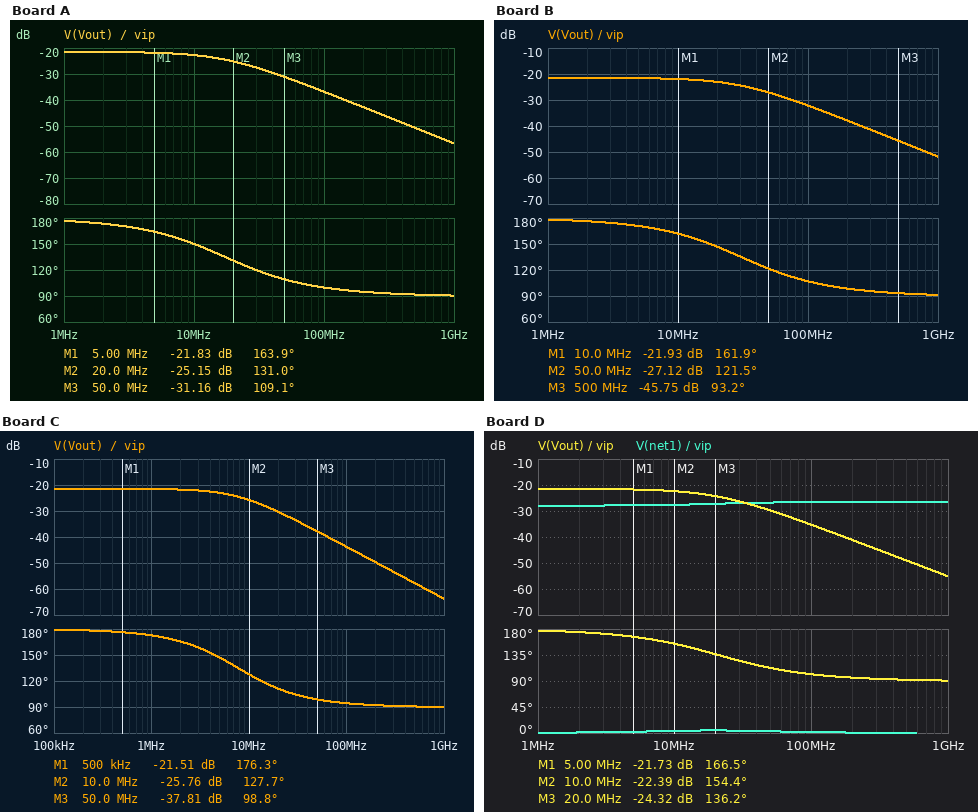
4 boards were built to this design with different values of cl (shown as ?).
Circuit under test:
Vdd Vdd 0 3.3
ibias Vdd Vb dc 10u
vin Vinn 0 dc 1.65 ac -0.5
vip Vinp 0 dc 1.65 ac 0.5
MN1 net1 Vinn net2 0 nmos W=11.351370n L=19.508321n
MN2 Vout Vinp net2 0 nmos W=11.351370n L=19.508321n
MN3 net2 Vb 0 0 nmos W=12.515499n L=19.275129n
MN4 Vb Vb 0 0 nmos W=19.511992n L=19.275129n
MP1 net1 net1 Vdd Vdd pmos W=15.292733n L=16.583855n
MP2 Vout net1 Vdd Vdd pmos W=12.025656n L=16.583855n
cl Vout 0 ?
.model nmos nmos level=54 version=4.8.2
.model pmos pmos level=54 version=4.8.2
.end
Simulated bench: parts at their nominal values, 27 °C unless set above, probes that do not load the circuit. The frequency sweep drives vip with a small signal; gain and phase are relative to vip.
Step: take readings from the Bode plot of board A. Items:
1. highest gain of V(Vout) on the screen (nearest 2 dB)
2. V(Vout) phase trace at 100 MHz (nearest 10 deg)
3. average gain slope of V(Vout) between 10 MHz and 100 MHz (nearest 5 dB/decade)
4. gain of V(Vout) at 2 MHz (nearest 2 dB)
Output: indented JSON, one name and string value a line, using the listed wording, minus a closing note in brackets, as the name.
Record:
{
  "highest gain of V(Vout) on the screen": "-22 dB",
  "V(Vout) phase trace at 100 MHz": "100 deg",
  "average gain slope of V(Vout) between 10 MHz and 100 MHz": "-15 dB/decade",
  "gain of V(Vout) at 2 MHz": "-22 dB"
}
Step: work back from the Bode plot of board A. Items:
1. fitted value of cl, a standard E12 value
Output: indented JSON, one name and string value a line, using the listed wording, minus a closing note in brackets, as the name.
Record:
{
  "fitted value of cl, a standard E12 value": "1.2 pF"
}
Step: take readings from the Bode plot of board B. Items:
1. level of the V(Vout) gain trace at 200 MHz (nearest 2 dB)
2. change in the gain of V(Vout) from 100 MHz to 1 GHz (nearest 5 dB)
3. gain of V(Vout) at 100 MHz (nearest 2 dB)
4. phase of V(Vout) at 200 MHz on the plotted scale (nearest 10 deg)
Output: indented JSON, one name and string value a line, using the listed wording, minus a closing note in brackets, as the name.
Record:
{
  "level of the V(Vout) gain trace at 200 MHz": "-38 dB",
  "change in the gain of V(Vout) from 100 MHz to 1 GHz": "-20 dB",
  "gain of V(Vout) at 100 MHz": "-32 dB",
  "phase of V(Vout) at 200 MHz on the plotted scale": "100 deg"
}
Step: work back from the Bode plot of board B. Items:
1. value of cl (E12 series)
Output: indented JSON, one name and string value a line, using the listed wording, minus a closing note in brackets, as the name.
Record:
{
  "value of cl": "680 fF"
}
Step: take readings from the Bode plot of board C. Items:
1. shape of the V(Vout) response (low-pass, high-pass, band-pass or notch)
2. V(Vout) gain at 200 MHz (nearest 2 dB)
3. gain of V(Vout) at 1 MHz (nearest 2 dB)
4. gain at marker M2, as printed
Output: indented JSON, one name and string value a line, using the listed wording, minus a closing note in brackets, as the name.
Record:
{
  "shape of the V(Vout) response": "low-pass",
  "V(Vout) gain at 200 MHz": "-50 dB",
  "gain of V(Vout) at 1 MHz": "-22 dB",
  "gain at marker M2, as printed": "-25.76 dB"
}
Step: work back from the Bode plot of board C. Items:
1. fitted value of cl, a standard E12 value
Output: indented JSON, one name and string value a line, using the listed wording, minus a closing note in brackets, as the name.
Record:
{
  "fitted value of cl, a standard E12 value": "2.7 pF"
}
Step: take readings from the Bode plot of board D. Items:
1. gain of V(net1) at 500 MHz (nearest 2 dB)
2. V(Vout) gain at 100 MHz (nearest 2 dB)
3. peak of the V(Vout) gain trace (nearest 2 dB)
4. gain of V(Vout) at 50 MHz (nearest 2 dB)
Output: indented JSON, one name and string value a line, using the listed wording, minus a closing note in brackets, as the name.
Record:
{
  "gain of V(net1) at 500 MHz": "-26 dB",
  "V(Vout) gain at 100 MHz": "-36 dB",
  "peak of the V(Vout) gain trace": "-22 dB",
  "gain of V(Vout) at 50 MHz": "-30 dB"
}
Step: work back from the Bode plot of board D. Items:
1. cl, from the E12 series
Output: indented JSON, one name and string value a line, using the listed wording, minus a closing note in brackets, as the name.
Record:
{
  "cl, from the E12 series": "1 pF"
}
